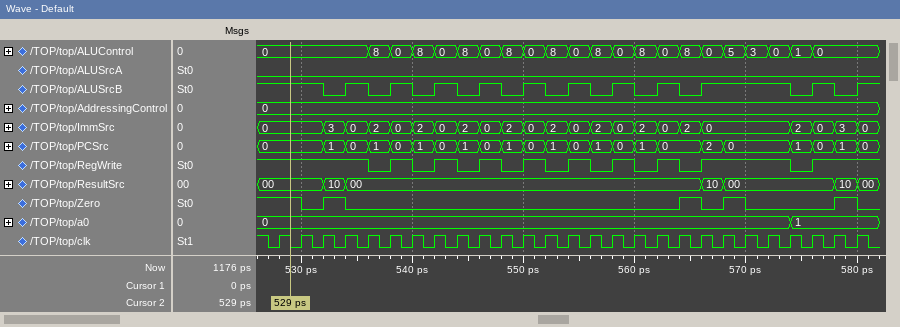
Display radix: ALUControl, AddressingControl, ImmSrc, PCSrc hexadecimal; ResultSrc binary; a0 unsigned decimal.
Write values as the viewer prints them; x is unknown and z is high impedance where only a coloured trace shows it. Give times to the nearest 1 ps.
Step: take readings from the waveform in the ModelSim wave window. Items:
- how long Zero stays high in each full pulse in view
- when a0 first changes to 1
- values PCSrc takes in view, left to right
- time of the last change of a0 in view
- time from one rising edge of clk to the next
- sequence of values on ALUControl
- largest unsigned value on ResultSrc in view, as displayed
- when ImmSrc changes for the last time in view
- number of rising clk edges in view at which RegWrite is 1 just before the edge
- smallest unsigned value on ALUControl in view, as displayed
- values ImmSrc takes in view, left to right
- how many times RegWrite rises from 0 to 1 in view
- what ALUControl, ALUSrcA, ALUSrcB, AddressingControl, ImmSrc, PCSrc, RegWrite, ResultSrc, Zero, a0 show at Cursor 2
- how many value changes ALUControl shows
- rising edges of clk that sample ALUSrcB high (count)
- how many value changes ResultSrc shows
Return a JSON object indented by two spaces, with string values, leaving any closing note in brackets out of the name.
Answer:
{
  "how long Zero stays high in each full pulse in view": "2 ps, 2 ps, 2 ps, 2 ps",
  "when a0 first changes to 1": "574 ps",
  "values PCSrc takes in view, left to right": "0, 1, 0, 1, 0, 1, 0, 1, 0, 1, 0, 1, 0, 1, 0, 1, 0, 2, 0, 1, 0, 1, 0",
  "time of the last change of a0 in view": "574 ps",
  "time from one rising edge of clk to the next": "2 ps",
  "sequence of values on ALUControl": "0, 8, 0, 8, 0, 8, 0, 8, 0, 8, 0, 8, 0, 8, 0, 8, 0, 5, 3, 0, 1, 0",
  "largest unsigned value on ResultSrc in view, as displayed": "10",
  "when ImmSrc changes for the last time in view": "580 ps",
  "number of rising clk edges in view at which RegWrite is 1 just before the edge": "18",
  "smallest unsigned value on ALUControl in view, as displayed": "0",
  "values ImmSrc takes in view, left to right": "0, 3, 0, 2, 0, 2, 0, 2, 0, 2, 0, 2, 0, 2, 0, 2, 0, 2, 0, 2, 0, 3, 0",
  "how many times RegWrite rises from 0 to 1 in view": "9",
  "what ALUControl, ALUSrcA, ALUSrcB, AddressingControl, ImmSrc, PCSrc, RegWrite, ResultSrc, Zero, a0 show at Cursor 2": "ALUControl=0, ALUSrcA=0, ALUSrcB=1, AddressingControl=0, ImmSrc=0, PCSrc=0, RegWrite=1, ResultSrc=00, Zero=1, a0=0",
  "how many value changes ALUControl shows": "21",
  "rising edges of clk that sample ALUSrcB high": "16",
  "how many value changes ResultSrc shows": "6"
}
